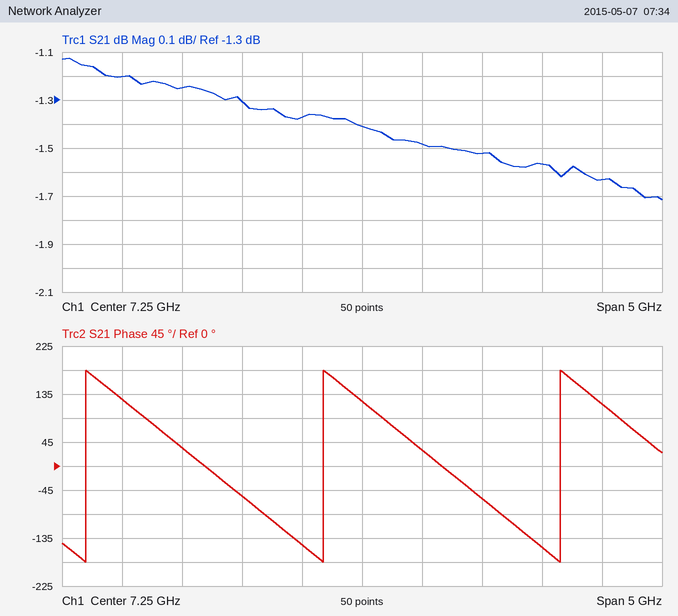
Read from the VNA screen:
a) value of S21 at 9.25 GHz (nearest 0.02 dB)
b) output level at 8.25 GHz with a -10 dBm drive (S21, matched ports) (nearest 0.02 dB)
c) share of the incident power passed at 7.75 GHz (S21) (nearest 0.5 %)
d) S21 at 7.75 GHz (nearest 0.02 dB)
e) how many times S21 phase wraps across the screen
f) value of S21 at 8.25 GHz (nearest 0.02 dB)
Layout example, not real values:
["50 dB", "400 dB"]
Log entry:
["-1.64 dB", "-11.52 dBm", "71.0 %", "-1.48 dB", "3", "-1.52 dB"]
